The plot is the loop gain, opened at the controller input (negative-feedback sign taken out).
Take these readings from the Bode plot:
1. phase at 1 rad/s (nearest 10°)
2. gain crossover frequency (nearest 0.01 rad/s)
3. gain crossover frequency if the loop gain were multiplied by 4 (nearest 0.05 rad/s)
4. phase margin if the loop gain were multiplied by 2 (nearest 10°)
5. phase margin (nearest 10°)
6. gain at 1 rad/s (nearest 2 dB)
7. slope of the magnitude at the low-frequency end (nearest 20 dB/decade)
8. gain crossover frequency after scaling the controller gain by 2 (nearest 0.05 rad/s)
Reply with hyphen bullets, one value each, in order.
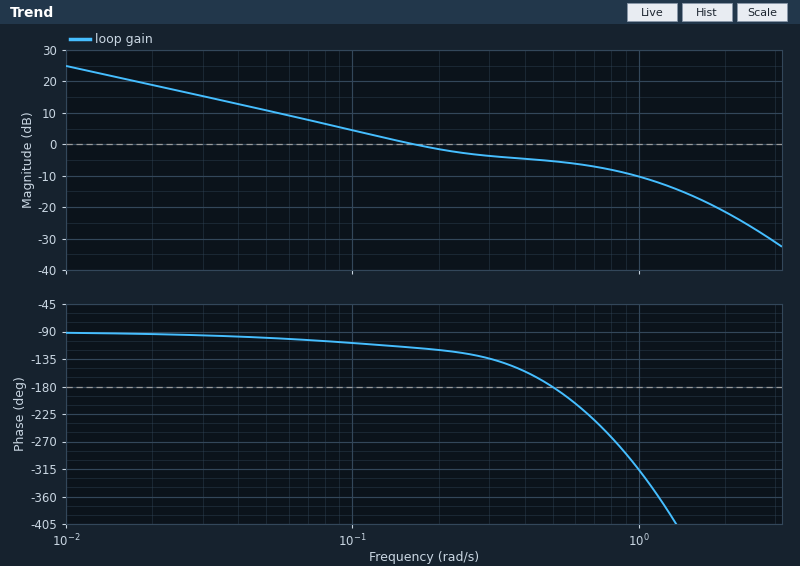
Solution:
- -320°
- 0.16 rad/s
- 1.15 rad/s
- -20°
- 60°
- -10 dB
- -20 dB/decade
- 0.60 rad/s
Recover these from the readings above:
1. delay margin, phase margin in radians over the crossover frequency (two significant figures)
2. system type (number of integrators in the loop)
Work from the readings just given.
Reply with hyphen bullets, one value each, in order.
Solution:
- 6.5 s
- 1
